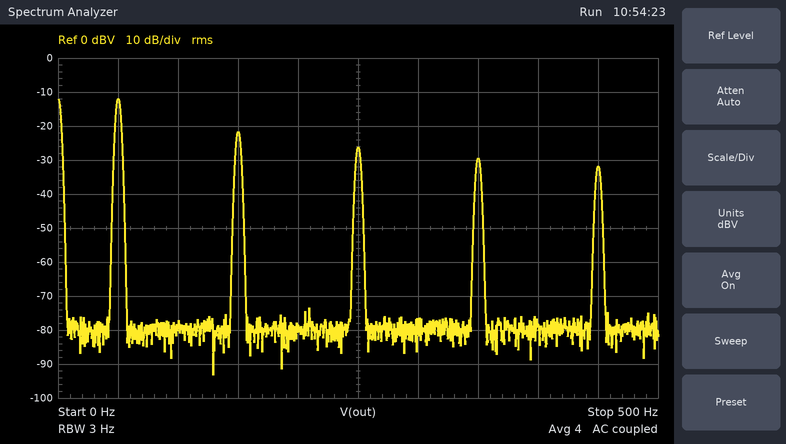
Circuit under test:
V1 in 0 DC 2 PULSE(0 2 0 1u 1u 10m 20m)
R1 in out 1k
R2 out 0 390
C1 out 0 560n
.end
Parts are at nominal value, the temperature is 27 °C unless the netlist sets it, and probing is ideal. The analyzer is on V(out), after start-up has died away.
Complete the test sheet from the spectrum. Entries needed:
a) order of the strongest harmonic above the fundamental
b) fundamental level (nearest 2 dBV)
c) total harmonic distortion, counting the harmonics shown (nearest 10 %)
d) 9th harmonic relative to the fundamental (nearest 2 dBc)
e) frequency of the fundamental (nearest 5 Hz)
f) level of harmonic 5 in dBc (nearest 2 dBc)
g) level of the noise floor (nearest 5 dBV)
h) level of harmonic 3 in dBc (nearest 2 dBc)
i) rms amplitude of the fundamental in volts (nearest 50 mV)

3
-12 dBV
40 %
-20 dBc
50 Hz
-14 dBc
-80 dBV
-10 dBc
250 mV
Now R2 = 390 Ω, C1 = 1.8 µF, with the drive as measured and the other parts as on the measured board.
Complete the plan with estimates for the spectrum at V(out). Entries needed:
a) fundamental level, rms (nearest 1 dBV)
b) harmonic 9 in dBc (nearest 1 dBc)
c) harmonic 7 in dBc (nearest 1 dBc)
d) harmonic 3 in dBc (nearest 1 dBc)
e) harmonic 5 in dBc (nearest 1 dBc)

-12 dBV
-24 dBc
-20 dBc
-10 dBc
-16 dBc
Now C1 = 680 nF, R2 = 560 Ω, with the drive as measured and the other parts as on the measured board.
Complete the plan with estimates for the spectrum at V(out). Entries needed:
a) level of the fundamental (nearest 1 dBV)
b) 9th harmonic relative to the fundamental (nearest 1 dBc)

-10 dBV
-21 dBc
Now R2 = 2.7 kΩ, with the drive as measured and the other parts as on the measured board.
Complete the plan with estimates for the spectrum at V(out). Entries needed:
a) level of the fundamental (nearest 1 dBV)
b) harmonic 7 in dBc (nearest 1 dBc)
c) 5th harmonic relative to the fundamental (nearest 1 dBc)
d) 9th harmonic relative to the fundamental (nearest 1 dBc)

-4 dBV
-19 dBc
-15 dBc
-23 dBc
